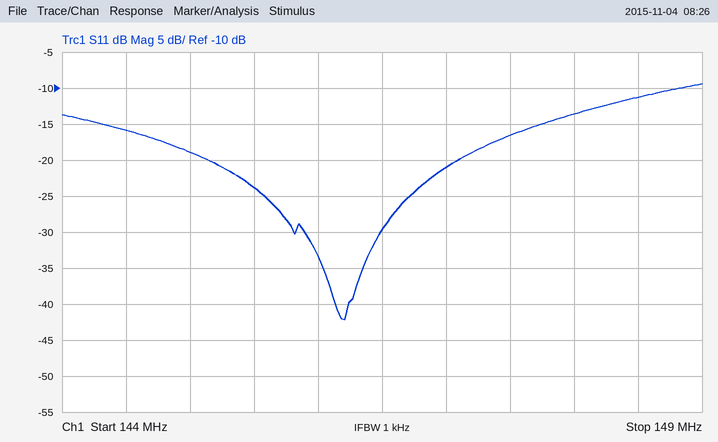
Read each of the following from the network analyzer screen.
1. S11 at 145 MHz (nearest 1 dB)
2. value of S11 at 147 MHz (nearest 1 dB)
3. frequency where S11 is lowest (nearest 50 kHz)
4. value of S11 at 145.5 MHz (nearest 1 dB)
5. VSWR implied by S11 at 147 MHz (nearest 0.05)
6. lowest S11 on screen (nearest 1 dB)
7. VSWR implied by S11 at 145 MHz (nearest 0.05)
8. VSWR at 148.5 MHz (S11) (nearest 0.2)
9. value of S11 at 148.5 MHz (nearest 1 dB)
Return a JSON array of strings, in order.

["-19 dB", "-21 dB", "146.20 MHz", "-24 dB", "1.20", "-42 dB", "1.25", "1.8", "-11 dB"]
